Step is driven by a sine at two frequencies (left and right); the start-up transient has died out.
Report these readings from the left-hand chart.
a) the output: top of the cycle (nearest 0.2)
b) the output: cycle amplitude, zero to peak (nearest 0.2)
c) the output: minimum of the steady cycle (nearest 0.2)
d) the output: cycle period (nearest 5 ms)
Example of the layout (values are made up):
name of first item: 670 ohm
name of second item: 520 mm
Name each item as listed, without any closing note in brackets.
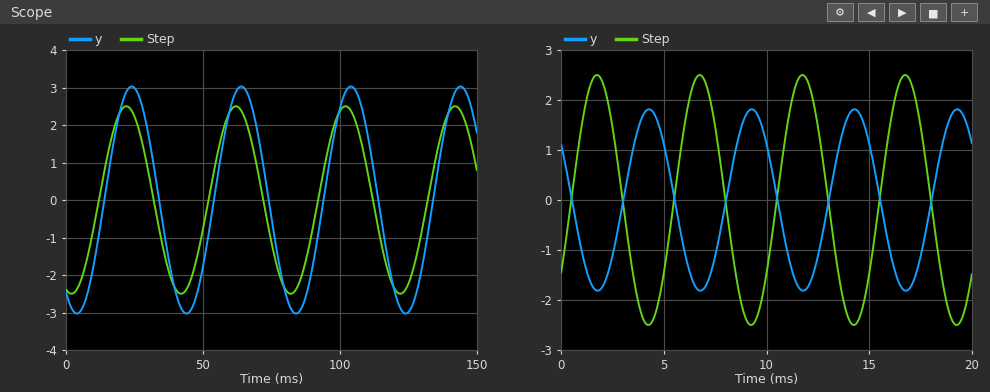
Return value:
the output: top of the cycle: 3.0
the output: cycle amplitude, zero to peak: 3.0
the output: minimum of the steady cycle: -3.0
the output: cycle period: 40 ms
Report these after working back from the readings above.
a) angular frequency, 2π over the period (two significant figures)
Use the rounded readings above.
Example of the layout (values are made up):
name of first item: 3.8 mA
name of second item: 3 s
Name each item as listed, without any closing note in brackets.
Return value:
angular frequency, 2π over the period: 0.16 rad/ms
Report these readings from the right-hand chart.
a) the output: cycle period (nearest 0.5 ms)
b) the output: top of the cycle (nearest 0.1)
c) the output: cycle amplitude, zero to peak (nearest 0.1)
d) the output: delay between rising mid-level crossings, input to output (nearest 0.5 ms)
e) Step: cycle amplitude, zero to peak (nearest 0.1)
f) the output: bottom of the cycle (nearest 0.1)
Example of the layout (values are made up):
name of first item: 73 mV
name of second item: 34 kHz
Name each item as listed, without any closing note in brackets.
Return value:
the output: cycle period: 5.0 ms
the output: top of the cycle: 1.8
the output: cycle amplitude, zero to peak: 1.8
the output: delay between rising mid-level crossings, input to output: 2.5 ms
Step: cycle amplitude, zero to peak: 2.5
the output: bottom of the cycle: -1.8
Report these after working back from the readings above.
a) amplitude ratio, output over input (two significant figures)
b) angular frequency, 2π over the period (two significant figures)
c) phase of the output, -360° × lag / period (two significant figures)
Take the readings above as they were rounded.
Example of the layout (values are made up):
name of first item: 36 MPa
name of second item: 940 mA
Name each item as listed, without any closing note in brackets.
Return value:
amplitude ratio, output over input: 0.72
angular frequency, 2π over the period: 1.3 rad/ms
phase of the output, -360° × lag / period: -180°
